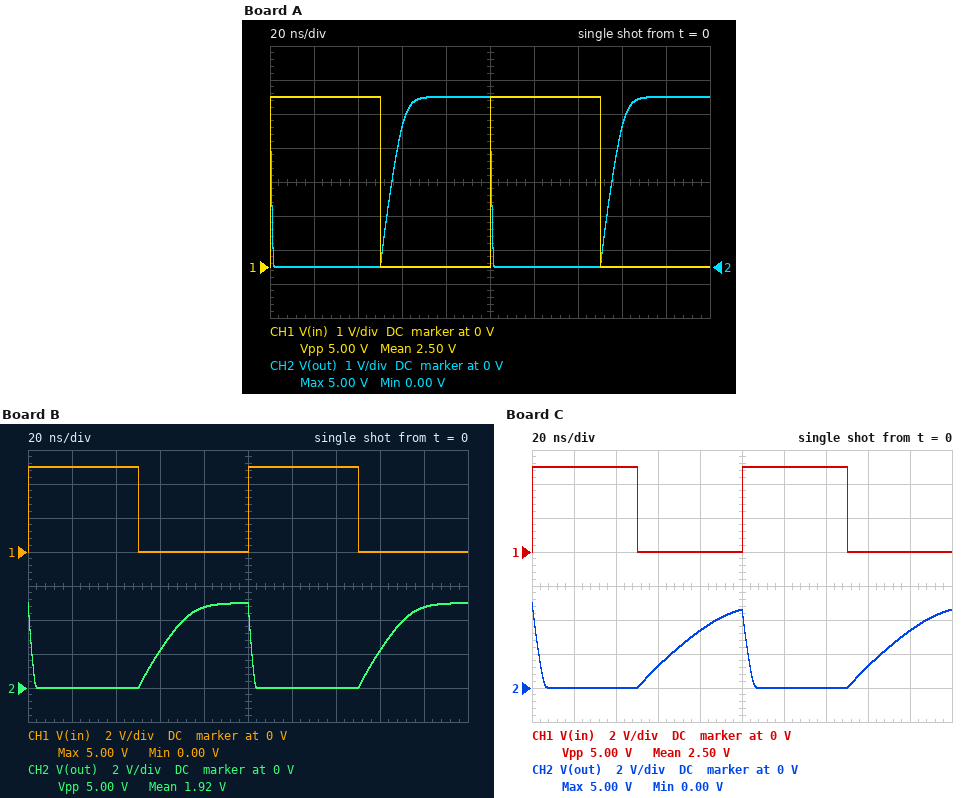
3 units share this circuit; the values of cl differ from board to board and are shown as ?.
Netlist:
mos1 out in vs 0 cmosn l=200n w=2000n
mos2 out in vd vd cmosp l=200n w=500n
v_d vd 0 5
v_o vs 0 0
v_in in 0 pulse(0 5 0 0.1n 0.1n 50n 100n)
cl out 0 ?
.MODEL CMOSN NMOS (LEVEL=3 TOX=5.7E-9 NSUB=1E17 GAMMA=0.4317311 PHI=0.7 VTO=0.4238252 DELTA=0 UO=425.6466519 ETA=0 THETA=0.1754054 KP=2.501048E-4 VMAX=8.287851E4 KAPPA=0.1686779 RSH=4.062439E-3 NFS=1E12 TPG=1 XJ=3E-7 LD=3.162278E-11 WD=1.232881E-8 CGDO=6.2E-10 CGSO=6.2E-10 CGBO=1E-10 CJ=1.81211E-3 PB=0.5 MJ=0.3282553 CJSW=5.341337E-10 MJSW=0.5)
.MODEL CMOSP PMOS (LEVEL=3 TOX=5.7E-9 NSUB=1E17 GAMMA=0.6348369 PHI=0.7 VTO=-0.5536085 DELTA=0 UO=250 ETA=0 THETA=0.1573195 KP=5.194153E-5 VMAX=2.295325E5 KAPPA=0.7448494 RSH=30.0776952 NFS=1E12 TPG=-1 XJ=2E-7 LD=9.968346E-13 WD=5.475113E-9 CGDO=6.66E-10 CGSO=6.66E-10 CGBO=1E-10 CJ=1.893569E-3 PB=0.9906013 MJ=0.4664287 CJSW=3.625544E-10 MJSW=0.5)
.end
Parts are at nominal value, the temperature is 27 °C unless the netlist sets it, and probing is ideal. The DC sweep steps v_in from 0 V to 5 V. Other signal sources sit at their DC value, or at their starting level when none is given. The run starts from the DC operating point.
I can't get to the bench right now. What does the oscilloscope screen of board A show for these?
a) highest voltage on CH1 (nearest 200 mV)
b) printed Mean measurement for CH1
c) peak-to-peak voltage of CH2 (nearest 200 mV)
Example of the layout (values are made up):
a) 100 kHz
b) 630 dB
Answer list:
a) 5.0 V
b) 2.50 V
c) 5.0 V
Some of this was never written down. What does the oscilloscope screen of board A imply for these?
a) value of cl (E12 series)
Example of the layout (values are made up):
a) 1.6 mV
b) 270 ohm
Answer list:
a) 820 fF
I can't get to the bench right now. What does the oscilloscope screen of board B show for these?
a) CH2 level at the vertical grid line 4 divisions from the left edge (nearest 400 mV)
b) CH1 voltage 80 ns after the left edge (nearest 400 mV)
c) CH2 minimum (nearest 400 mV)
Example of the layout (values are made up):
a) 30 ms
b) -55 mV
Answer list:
a) 4.8 V
b) 0 V
c) 0 V
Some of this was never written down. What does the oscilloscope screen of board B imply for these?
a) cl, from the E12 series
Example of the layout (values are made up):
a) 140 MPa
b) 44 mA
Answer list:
a) 1.8 pF
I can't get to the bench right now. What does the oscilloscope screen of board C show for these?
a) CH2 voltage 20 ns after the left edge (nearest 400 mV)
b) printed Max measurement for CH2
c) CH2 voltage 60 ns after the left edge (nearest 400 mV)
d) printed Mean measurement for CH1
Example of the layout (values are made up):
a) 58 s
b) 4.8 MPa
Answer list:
a) 0 V
b) 5.00 V
c) 1.2 V
d) 2.50 V
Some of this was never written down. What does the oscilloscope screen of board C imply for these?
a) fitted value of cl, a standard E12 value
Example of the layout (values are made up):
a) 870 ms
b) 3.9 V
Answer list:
a) 3.3 pF
